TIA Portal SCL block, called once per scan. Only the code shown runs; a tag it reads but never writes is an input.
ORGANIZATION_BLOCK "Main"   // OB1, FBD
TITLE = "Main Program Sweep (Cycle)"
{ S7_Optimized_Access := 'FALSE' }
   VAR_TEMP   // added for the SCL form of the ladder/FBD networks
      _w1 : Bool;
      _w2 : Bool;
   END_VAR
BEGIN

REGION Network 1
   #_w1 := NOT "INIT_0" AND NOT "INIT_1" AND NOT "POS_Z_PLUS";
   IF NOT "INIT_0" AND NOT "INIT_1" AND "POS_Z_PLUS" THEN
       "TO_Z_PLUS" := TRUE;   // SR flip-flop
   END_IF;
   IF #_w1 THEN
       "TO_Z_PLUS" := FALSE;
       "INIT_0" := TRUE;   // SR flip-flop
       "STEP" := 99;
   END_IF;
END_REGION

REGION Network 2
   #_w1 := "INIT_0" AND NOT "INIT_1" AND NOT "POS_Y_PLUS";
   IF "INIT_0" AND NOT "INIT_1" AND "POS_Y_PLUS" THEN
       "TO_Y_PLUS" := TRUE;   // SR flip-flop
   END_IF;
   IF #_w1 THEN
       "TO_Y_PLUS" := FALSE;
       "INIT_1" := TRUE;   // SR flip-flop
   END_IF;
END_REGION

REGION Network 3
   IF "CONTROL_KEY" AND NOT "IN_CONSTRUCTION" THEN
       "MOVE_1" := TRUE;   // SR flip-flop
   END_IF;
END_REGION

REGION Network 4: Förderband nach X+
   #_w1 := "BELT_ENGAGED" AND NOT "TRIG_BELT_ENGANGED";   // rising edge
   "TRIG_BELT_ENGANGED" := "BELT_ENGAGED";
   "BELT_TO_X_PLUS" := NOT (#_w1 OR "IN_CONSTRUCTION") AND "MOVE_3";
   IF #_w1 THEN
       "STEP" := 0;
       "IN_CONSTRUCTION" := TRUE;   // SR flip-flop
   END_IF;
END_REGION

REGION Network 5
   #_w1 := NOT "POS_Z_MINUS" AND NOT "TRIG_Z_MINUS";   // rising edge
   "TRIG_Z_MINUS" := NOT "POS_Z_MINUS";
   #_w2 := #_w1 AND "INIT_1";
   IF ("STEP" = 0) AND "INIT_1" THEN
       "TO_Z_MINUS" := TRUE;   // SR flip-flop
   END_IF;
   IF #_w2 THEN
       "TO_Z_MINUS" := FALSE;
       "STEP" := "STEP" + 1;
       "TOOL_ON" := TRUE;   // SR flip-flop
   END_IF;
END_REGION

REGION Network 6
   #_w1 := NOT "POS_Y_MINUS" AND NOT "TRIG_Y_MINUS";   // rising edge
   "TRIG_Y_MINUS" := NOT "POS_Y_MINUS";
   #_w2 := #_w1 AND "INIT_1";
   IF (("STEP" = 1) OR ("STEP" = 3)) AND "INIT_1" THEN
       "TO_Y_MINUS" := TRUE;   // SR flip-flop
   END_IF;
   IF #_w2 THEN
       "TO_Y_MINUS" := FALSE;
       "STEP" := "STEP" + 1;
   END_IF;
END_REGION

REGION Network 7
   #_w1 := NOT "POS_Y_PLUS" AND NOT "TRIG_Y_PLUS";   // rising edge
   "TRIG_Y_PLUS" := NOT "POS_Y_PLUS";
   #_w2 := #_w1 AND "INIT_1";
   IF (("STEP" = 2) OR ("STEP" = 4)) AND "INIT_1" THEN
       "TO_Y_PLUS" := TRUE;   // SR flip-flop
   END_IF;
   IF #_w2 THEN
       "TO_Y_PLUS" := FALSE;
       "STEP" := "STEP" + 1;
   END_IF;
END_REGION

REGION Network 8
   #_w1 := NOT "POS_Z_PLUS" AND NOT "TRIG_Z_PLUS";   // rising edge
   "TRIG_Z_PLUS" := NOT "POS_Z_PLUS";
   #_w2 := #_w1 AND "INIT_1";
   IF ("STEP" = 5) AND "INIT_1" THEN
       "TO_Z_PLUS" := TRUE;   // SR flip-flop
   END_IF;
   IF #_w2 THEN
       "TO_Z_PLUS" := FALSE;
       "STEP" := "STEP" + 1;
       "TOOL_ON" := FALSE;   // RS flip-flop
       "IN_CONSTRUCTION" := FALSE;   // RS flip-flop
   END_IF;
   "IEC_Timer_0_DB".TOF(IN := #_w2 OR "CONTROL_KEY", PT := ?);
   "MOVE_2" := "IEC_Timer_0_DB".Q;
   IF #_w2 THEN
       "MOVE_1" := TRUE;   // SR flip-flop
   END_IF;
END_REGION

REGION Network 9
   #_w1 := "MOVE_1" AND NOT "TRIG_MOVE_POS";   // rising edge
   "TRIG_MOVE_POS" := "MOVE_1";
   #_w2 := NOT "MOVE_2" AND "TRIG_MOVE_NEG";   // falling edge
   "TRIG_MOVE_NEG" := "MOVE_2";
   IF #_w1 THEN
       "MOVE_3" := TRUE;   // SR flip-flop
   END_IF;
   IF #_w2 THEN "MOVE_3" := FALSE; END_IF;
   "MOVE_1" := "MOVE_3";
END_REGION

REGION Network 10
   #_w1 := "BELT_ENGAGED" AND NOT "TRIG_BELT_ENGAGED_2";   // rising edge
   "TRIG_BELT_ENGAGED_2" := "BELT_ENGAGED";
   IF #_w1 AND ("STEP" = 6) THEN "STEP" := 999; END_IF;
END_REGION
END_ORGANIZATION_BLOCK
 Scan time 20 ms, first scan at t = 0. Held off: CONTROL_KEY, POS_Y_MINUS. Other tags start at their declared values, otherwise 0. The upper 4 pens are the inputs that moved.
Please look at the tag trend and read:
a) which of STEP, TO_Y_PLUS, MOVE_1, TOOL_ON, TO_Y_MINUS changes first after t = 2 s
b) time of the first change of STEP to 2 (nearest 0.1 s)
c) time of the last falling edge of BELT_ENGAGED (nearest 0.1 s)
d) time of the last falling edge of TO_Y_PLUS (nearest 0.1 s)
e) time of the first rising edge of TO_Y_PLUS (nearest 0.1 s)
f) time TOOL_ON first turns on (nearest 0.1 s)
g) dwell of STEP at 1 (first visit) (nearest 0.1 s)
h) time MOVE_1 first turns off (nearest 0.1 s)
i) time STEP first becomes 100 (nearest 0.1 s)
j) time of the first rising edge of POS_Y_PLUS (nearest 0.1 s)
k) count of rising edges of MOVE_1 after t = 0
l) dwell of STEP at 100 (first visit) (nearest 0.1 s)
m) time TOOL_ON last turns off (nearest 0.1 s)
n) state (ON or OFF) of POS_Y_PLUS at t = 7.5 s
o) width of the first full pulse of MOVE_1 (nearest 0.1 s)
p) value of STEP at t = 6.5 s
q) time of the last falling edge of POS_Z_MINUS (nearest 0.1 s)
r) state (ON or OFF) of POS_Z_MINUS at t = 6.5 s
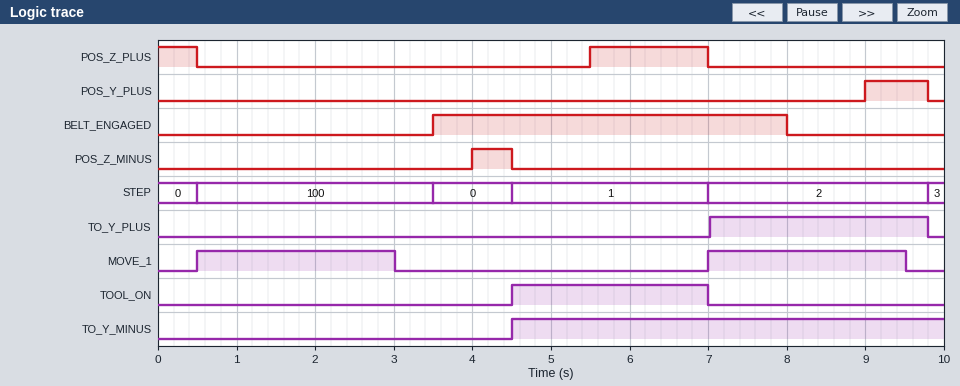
MOVE_1
7.0 s
8.0 s
9.8 s
7.0 s
4.5 s
2.5 s
3.0 s
0.5 s
9.0 s
2
3.0 s
7.0 s
OFF
2.5 s
1
4.5 s
OFF
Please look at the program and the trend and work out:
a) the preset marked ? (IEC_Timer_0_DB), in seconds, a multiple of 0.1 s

2.5 s
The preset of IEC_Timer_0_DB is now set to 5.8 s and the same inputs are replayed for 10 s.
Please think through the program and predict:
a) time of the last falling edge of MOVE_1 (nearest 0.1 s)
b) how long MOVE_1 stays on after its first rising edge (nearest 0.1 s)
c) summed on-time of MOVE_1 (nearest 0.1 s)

6.3 s
5.8 s
8.8 s
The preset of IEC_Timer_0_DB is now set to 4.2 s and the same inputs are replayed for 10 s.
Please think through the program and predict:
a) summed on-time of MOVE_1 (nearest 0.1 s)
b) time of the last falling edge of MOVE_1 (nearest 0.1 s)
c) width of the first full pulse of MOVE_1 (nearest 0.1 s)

7.2 s
4.7 s
4.2 s
